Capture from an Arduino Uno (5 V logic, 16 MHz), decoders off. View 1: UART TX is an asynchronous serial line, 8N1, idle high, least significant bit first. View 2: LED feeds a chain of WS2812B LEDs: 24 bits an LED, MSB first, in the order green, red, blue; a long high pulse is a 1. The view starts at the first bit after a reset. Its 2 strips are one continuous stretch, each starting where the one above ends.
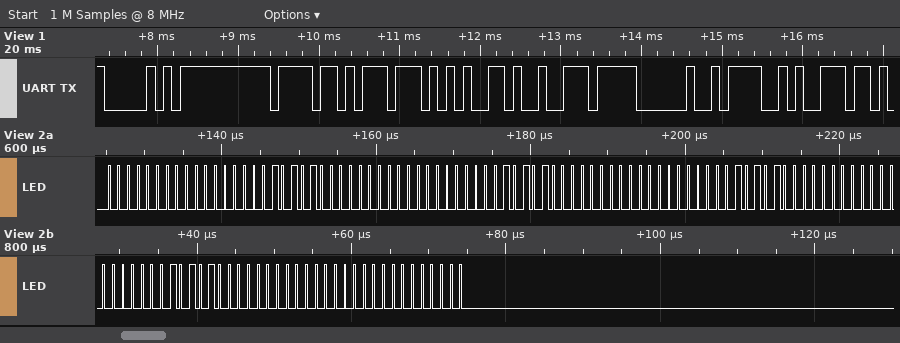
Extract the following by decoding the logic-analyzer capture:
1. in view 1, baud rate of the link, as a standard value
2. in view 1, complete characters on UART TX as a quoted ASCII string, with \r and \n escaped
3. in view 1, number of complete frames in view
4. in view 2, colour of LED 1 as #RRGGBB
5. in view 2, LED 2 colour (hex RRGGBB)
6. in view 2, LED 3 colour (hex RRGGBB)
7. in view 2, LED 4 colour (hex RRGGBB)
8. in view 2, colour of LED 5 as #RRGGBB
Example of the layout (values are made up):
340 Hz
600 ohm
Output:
9600 baud
"Power On"
8
#000054
#000054
#000054
#000054
#000000
